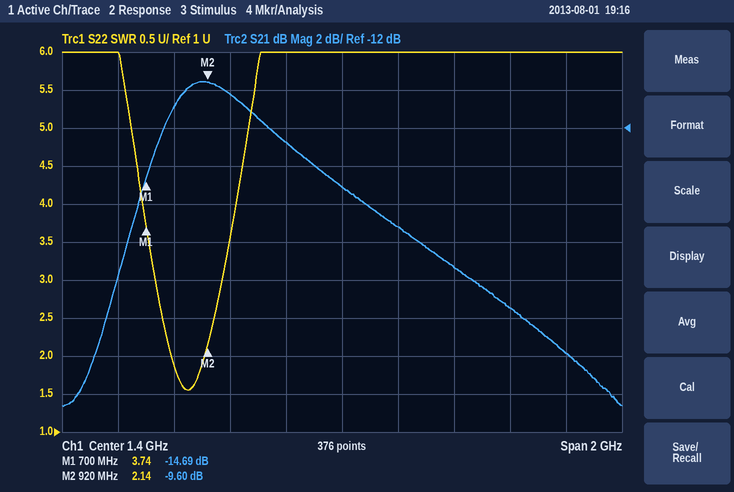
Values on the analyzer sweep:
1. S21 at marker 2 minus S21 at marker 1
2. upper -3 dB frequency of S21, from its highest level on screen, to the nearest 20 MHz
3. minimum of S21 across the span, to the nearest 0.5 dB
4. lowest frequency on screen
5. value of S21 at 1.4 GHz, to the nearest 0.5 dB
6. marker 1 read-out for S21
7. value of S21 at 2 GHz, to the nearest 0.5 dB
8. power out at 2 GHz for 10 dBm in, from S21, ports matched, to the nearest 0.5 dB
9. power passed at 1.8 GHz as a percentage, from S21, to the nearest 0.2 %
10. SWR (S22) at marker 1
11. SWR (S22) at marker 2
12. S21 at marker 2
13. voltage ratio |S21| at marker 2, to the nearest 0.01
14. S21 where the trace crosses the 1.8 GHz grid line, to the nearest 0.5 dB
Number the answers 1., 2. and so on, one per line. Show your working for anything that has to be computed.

1. -9.6 − (-14.69) = 5.09 dB
2. 1.18 GHz
3. -26.5 dB
4. 400 MHz
5. -15.0 dB
6. -14.69 dB
7. -21.5 dB
8. 10 dBm + (-21.5 dB) = -11.5 dBm
9. 10^(-19.5/10) ≈ 1.12 %, so 1.2 % to the nearest 0.2 %
10. 3.74
11. 2.14
12. -9.60 dB
13. 10^(-9.6/20) ≈ 0.33
14. -19.5 dB
